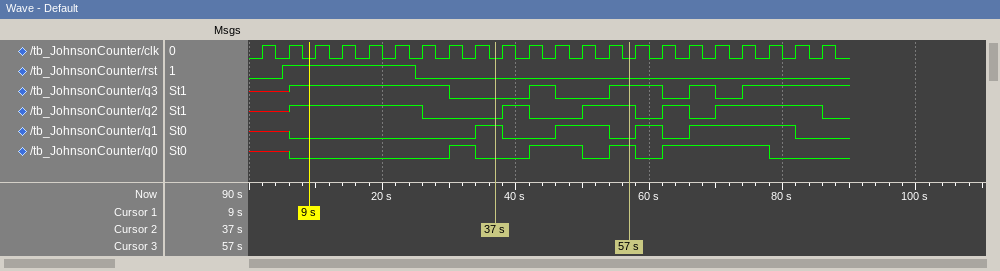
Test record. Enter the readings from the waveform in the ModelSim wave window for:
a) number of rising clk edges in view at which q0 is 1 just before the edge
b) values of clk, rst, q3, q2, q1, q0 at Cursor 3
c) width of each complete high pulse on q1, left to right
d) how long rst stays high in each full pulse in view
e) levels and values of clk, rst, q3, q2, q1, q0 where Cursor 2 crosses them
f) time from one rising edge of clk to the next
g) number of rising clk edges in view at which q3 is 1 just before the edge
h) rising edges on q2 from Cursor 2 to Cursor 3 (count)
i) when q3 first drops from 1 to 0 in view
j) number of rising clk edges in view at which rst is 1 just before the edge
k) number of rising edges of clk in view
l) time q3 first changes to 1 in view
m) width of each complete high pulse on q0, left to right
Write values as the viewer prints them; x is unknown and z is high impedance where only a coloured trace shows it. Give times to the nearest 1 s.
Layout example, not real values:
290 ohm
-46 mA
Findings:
8
clk=0, rst=0, q3=1, q2=1, q1=0, q0=1
4 s, 8 s, 4 s, 16 s
20 s
clk=0, rst=0, q3=0, q2=0, q1=1, q0=0
4 s
13
2
30 s
5
22
6 s
4 s, 8 s, 4 s, 16 s
